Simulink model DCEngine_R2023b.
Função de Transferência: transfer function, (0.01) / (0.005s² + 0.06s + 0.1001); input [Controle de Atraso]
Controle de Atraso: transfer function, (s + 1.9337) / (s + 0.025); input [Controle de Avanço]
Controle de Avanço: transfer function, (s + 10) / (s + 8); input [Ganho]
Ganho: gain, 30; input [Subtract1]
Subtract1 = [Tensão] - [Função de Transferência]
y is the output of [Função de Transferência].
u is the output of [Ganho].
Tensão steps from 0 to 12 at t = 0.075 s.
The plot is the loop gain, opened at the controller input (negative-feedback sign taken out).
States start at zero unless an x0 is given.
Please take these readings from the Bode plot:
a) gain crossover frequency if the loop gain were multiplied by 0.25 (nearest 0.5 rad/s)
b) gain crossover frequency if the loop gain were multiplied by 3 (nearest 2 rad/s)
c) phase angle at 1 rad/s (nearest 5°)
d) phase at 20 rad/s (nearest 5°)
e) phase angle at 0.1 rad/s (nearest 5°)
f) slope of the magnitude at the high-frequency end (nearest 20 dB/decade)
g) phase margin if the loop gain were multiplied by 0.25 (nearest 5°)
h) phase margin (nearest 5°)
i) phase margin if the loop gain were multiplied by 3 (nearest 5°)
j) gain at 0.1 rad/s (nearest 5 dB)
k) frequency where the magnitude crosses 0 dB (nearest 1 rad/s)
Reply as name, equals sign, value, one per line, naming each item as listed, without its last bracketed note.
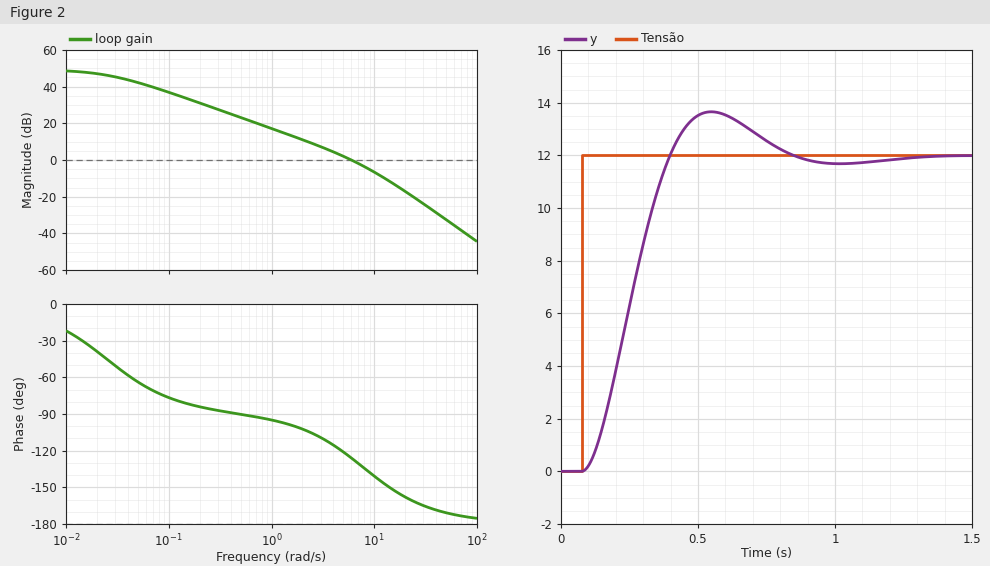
gain crossover frequency if the loop gain were multiplied by 0.25 = 2.0 rad/s
gain crossover frequency if the loop gain were multiplied by 3 = 12 rad/s
phase angle at 1 rad/s = -95°
phase at 20 rad/s = -160°
phase angle at 0.1 rad/s = -75°
slope of the magnitude at the high-frequency end = -40 dB/decade
phase margin if the loop gain were multiplied by 0.25 = 80°
phase margin = 55°
phase margin if the loop gain were multiplied by 3 = 35°
gain at 0.1 rad/s = 35 dB
frequency where the magnitude crosses 0 dB = 6 rad/s
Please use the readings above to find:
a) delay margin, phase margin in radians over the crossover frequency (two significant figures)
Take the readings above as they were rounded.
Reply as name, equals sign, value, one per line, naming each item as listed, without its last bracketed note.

delay margin, phase margin in radians over the crossover frequency = 0.16 s
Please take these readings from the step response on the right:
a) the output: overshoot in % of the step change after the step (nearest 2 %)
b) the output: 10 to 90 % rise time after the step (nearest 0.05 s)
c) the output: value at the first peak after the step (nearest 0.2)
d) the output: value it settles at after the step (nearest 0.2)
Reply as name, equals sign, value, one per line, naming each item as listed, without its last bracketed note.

the output: overshoot in % of the step change after the step = 14 %
the output: 10 to 90 % rise time after the step = 0.20 s
the output: value at the first peak after the step = 13.6
the output: value it settles at after the step = 12.0
